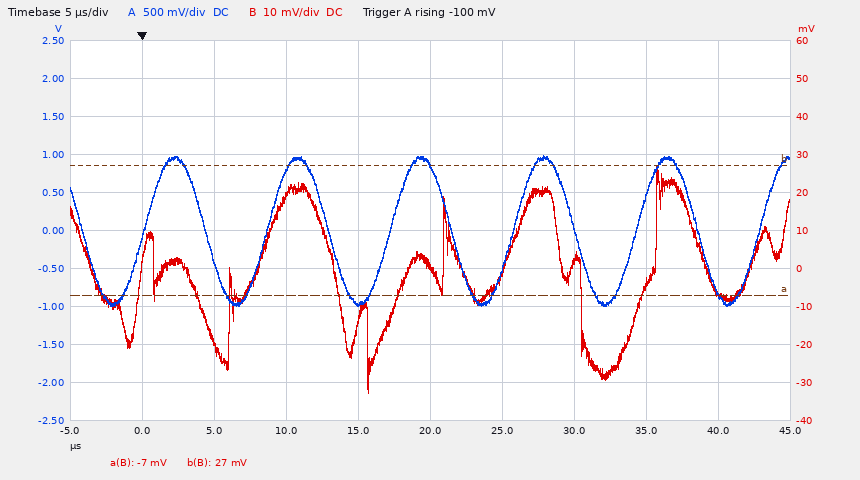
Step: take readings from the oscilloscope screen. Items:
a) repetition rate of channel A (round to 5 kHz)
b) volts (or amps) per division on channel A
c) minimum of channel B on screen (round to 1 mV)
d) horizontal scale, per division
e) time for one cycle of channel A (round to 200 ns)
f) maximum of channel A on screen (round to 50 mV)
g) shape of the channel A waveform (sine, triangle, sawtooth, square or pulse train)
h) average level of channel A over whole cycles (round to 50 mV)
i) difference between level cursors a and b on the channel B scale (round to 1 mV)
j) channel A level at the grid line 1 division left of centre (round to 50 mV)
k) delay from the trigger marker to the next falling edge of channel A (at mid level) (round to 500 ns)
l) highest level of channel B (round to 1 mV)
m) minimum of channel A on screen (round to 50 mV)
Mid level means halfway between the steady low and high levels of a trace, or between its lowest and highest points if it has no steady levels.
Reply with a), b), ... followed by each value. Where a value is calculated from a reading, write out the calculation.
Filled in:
a) 1 / 8.6 µs ≈ 116 kHz, so 115 kHz to the nearest 5 kHz
b) 500 mV
c) -33 mV
d) 5 µs
e) 8.6 µs
f) 1.00 V
g) sine
h) (1.00 V + (-1.00 V)) / 2 ≈ 0 mV
i) 34 mV
j) -950 mV
k) 4.5 µs
l) 27 mV
m) -1.00 V
